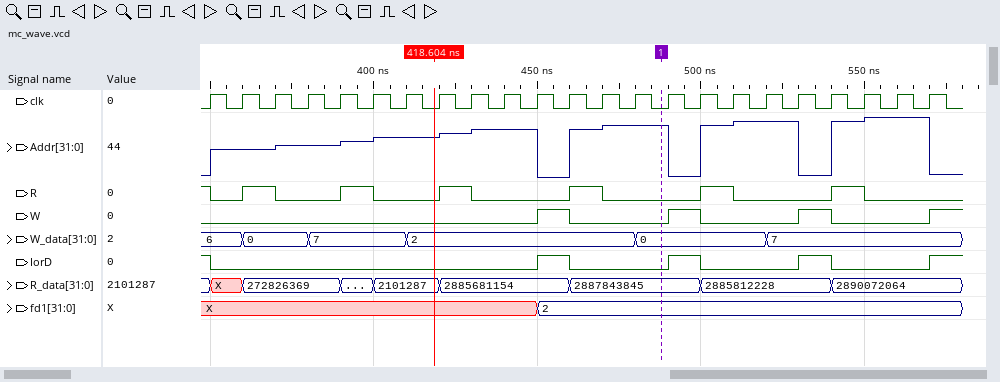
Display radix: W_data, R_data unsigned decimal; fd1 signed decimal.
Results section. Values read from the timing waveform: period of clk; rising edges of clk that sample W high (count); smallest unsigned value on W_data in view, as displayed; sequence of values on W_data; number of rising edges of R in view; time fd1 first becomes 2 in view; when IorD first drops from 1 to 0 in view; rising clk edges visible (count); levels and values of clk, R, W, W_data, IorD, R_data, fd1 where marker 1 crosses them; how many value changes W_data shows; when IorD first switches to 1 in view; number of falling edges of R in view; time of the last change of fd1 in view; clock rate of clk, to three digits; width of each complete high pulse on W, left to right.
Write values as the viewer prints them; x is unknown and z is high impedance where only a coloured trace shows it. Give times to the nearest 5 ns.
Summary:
10 ns
3
0
6, 0, 7, 2, 0, 7
6
450 ns
350 ns
23
clk=0, R=0, W=0, W_data=0, IorD=0, R_data=2887843845, fd1=2
5
450 ns
7
450 ns
100 MHz
10 ns, 10 ns, 10 ns
